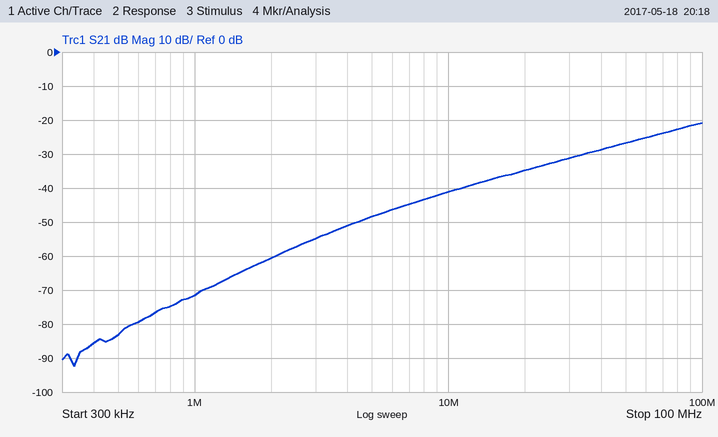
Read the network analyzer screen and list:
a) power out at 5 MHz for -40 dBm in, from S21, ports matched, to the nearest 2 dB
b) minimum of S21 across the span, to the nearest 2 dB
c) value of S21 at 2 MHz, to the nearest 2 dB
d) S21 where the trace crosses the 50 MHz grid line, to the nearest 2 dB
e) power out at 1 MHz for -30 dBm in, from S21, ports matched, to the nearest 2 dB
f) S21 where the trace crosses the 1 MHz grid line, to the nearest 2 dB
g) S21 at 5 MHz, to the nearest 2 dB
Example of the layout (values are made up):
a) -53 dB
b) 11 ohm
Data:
a) -88 dBm
b) -92 dB
c) -60 dB
d) -26 dB
e) -102 dBm
f) -72 dB
g) -48 dB
